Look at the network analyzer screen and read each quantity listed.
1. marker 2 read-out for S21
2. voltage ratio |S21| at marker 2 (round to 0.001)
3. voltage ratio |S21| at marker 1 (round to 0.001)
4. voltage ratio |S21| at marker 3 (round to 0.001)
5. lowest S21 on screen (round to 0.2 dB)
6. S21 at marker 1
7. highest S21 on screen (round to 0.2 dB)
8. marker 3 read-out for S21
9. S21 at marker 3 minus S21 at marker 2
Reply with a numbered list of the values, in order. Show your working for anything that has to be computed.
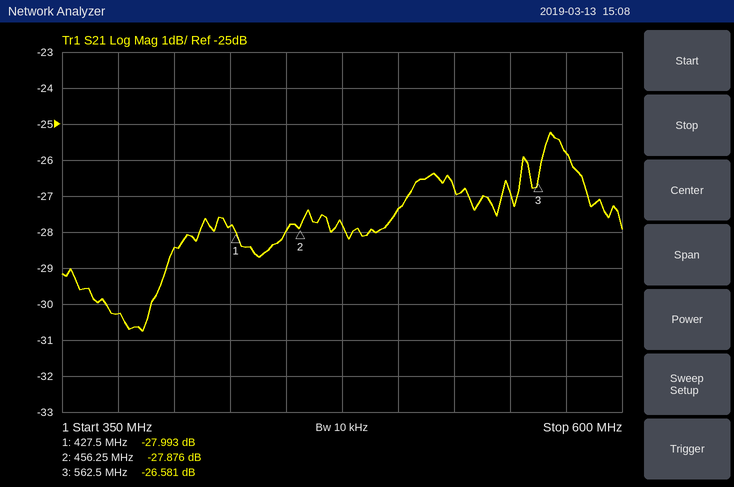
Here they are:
1. -27.876 dB
2. 10^(-27.876/20) ≈ 0.040
3. 10^(-27.993/20) ≈ 0.040
4. 10^(-26.581/20) ≈ 0.047
5. -30.8 dB
6. -27.993 dB
7. -25.2 dB
8. -26.581 dB
9. -26.581 − (-27.876) = 1.295 dB
